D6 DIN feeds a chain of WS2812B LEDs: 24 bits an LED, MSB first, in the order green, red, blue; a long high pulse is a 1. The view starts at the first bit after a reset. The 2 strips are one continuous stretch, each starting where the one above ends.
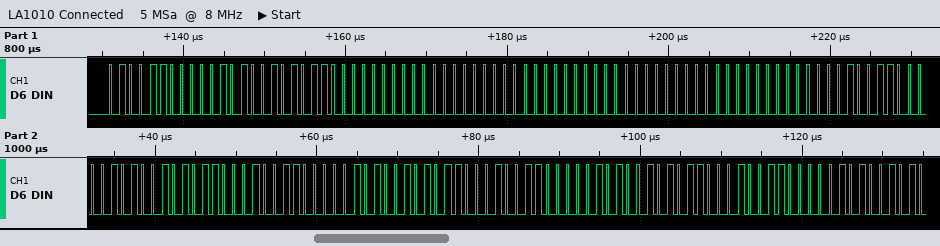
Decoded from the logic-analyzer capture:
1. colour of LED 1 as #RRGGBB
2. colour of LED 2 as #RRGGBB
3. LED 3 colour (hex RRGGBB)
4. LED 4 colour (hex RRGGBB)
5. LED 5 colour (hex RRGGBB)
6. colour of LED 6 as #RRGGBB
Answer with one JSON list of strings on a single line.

["#144CAC", "#000000", "#000000", "#144CAC", "#144CAC", "#144CAC"]
